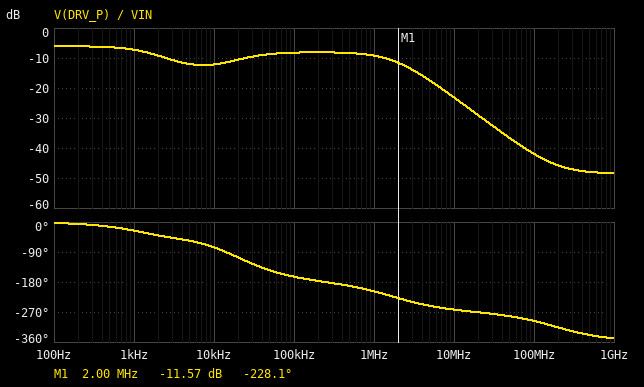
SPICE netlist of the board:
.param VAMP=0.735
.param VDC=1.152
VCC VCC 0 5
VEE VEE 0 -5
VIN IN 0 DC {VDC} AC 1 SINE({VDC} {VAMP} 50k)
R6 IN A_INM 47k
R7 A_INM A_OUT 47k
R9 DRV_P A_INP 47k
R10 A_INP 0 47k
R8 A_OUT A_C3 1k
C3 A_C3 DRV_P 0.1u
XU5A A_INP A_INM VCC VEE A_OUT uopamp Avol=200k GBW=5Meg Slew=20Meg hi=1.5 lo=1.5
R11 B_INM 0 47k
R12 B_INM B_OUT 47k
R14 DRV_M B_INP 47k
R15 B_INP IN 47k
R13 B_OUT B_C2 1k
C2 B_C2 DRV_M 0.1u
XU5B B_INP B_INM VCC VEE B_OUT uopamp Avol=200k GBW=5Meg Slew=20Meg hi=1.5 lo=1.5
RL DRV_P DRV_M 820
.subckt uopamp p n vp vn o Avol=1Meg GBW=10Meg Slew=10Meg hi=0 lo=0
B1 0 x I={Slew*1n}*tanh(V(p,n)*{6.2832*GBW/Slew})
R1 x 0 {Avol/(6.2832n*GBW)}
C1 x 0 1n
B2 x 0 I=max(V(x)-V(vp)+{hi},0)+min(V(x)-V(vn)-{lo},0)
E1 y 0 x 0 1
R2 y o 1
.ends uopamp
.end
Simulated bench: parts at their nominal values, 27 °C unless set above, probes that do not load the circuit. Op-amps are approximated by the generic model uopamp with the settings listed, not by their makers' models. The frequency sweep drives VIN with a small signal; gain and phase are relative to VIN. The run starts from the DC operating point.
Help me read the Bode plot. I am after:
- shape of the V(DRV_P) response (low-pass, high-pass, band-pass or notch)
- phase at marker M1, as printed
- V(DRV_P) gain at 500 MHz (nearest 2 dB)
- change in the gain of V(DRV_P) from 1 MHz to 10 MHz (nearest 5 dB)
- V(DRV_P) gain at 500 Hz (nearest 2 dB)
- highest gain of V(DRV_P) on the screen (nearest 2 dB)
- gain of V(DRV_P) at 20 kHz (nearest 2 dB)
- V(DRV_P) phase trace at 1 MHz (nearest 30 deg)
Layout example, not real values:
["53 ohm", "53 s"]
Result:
["low-pass", "-228.1 deg", "-48 dB", "-15 dB", "-6 dB", "-6 dB", "-10 dB", "-210 deg"]
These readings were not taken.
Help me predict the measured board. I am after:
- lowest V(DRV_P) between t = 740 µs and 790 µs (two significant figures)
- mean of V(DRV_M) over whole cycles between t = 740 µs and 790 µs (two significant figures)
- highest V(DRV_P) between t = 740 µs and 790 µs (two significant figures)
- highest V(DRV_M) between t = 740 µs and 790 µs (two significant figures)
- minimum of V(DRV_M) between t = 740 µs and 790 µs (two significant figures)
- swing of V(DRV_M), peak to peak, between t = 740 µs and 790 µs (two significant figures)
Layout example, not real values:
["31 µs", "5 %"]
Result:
["300 mV", "580 mV", "840 mV", "990 mV", "170 mV", "820 mV"]
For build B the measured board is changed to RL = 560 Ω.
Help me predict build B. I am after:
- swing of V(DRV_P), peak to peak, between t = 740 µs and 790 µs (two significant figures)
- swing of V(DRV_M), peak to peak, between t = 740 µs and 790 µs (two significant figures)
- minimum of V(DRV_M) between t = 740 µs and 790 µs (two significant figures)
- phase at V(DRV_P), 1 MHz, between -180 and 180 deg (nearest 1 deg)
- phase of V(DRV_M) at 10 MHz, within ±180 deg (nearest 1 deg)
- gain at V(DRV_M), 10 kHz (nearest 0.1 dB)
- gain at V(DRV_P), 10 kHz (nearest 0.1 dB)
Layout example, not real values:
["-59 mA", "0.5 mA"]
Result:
["400 mV", "650 mV", "250 mV", "155 deg", "-73 deg", "-2.5 dB", "-10.8 dB"]
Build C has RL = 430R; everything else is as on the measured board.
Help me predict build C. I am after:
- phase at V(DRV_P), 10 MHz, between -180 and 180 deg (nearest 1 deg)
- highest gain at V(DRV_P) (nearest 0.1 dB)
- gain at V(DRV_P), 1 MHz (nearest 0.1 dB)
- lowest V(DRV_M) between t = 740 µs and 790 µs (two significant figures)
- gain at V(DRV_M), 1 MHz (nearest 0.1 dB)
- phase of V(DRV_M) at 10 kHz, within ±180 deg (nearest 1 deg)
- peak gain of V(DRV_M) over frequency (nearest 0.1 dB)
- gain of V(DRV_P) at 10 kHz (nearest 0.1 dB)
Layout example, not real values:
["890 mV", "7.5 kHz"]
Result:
["96 deg", "-6.0 dB", "-14.7 dB", "290 mV", "-13.8 dB", "-12 deg", "-3.0 dB", "-9.7 dB"]
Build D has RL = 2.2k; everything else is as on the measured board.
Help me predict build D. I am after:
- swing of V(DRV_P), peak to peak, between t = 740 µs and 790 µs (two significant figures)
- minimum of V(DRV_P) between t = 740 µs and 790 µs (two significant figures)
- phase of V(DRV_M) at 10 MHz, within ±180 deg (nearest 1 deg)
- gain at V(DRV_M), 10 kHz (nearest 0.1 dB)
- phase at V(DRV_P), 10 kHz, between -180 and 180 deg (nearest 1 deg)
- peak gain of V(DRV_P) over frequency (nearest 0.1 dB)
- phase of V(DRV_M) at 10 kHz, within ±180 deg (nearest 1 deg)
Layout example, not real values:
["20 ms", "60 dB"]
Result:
["1.5 V", "-170 mV", "-80 deg", "3.7 dB", "-151 deg", "0.5 dB", "-1 deg"]
